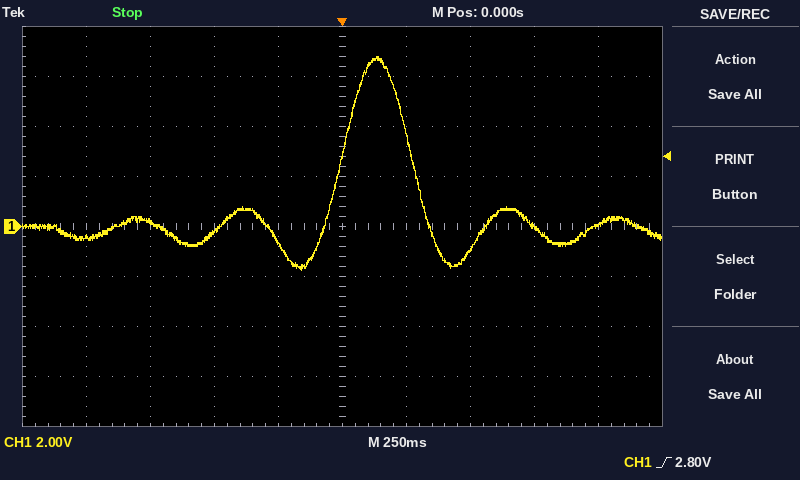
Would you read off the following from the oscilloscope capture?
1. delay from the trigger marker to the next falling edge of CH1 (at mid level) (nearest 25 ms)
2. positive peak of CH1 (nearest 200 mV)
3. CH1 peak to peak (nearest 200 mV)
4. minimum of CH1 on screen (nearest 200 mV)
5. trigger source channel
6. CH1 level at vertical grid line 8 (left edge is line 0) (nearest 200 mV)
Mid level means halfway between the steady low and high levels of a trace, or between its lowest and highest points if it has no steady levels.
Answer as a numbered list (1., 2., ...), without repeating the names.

1. 275 ms
2. 6.8 V
3. 8.6 V
4. -1.8 V
5. CH1
6. 0.0 V
